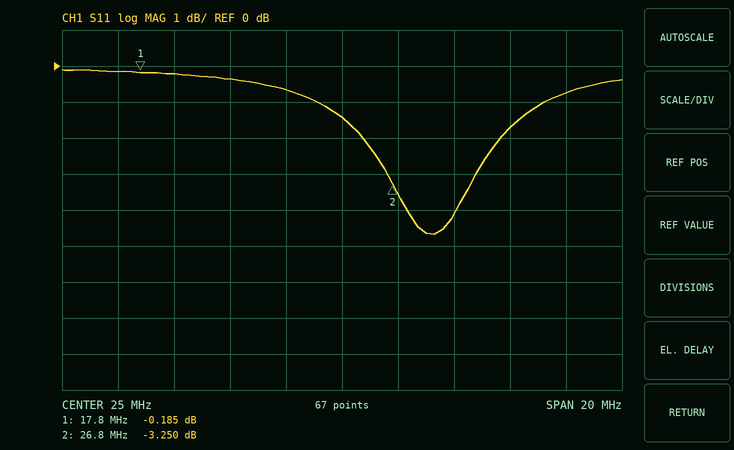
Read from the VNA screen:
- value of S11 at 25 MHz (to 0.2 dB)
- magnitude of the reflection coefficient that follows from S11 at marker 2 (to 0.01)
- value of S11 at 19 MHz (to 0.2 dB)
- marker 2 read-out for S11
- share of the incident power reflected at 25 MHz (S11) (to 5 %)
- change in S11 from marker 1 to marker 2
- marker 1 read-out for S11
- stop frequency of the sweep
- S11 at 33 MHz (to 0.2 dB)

-1.4 dB
0.69
-0.2 dB
-3.250 dB
70 %
-3.065 dB
-0.185 dB
35 MHz
-0.8 dB
